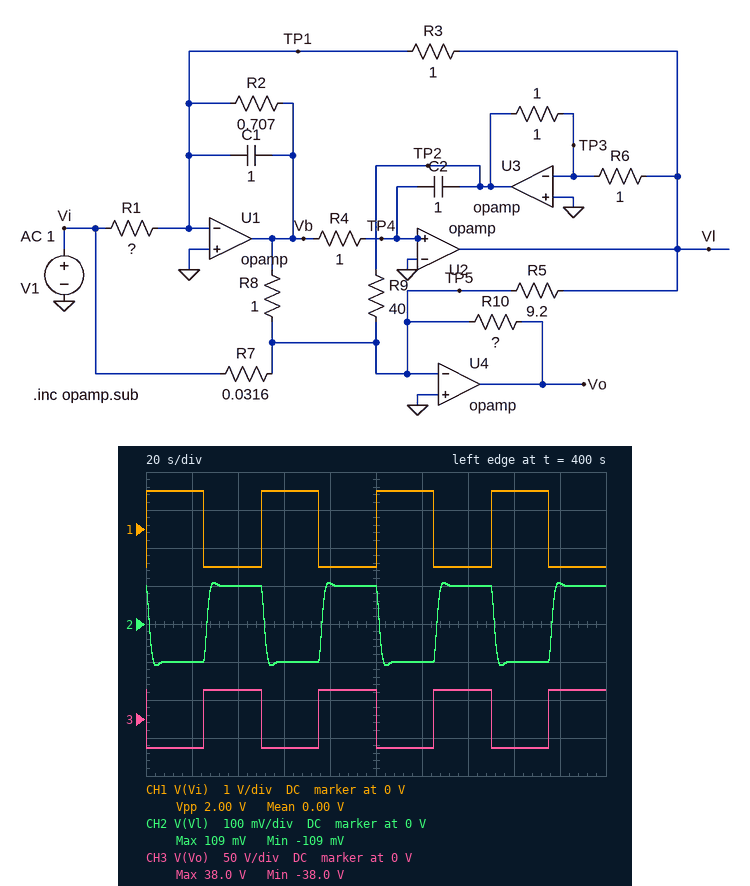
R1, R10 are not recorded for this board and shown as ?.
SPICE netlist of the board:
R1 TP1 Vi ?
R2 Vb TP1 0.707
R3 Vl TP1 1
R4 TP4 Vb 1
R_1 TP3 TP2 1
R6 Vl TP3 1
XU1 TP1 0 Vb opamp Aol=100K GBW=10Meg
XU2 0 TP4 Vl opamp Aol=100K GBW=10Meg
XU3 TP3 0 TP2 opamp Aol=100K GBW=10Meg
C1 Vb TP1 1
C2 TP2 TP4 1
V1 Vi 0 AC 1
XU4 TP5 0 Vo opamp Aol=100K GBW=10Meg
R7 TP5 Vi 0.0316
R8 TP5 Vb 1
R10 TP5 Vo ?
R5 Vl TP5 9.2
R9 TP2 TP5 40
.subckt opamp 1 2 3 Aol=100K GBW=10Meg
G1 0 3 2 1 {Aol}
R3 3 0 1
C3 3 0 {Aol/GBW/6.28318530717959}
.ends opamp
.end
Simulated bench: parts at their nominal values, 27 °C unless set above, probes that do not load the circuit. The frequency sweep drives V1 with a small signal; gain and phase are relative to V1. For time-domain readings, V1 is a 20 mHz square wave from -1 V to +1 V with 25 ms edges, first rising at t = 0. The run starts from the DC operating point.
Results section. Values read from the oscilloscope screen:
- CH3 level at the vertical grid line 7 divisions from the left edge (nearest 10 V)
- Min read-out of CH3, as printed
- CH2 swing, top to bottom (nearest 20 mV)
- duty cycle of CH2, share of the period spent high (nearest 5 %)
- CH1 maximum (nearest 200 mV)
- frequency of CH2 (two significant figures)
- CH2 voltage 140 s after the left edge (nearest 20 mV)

40 V
-38.0 V
220 mV
50 %
1.0 V
20 mHz
100 mV
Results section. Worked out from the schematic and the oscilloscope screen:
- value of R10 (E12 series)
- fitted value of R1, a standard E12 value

1.2 Ω
10 Ω
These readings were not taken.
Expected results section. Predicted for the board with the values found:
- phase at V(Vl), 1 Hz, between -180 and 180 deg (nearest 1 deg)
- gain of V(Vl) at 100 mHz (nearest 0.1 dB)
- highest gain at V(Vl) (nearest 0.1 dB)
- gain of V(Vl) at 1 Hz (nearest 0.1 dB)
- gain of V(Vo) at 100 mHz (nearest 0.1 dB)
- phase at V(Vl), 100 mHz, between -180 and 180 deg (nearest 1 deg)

13 deg
-20.6 dB
-20.0 dB
-51.9 dB
31.6 dB
124 deg
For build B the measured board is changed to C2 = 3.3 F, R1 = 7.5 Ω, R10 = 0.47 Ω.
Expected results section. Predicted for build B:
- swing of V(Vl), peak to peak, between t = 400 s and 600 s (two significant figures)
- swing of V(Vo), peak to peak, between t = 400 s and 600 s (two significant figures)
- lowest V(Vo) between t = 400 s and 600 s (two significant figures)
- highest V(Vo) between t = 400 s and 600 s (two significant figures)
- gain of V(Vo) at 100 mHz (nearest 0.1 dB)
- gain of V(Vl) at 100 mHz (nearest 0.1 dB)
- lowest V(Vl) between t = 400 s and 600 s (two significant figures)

270 mV
30 V
-15 V
15 V
23.4 dB
-26.9 dB
-130 mV
